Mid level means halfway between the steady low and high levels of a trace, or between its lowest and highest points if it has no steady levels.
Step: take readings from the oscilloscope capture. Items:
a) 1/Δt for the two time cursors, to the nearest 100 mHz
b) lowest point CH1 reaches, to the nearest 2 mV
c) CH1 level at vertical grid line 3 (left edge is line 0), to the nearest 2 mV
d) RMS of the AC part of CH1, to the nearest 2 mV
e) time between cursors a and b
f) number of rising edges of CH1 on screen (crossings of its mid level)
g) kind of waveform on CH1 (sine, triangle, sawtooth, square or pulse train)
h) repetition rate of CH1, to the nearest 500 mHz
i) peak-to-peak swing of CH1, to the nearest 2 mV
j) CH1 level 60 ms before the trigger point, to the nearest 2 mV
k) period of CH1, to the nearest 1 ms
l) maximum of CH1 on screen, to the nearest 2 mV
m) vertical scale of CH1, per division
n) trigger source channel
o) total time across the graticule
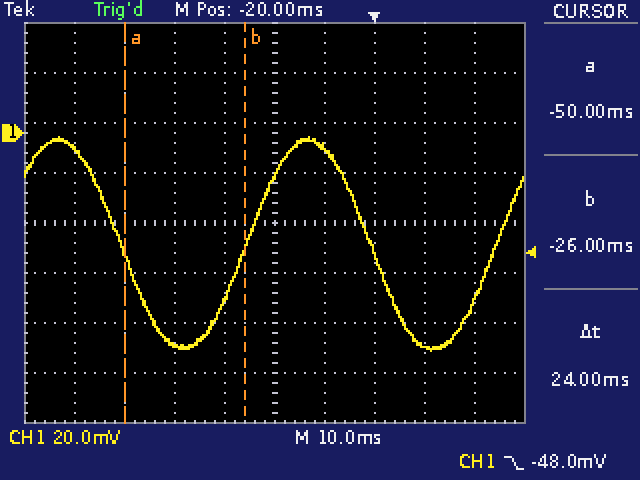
41.7 Hz
-88 mV
-84 mV
30 mV
24 ms
2
sine
20.0 Hz
86 mV
-6 mV
50 ms
-2 mV
20 mV
CH1
100 ms
